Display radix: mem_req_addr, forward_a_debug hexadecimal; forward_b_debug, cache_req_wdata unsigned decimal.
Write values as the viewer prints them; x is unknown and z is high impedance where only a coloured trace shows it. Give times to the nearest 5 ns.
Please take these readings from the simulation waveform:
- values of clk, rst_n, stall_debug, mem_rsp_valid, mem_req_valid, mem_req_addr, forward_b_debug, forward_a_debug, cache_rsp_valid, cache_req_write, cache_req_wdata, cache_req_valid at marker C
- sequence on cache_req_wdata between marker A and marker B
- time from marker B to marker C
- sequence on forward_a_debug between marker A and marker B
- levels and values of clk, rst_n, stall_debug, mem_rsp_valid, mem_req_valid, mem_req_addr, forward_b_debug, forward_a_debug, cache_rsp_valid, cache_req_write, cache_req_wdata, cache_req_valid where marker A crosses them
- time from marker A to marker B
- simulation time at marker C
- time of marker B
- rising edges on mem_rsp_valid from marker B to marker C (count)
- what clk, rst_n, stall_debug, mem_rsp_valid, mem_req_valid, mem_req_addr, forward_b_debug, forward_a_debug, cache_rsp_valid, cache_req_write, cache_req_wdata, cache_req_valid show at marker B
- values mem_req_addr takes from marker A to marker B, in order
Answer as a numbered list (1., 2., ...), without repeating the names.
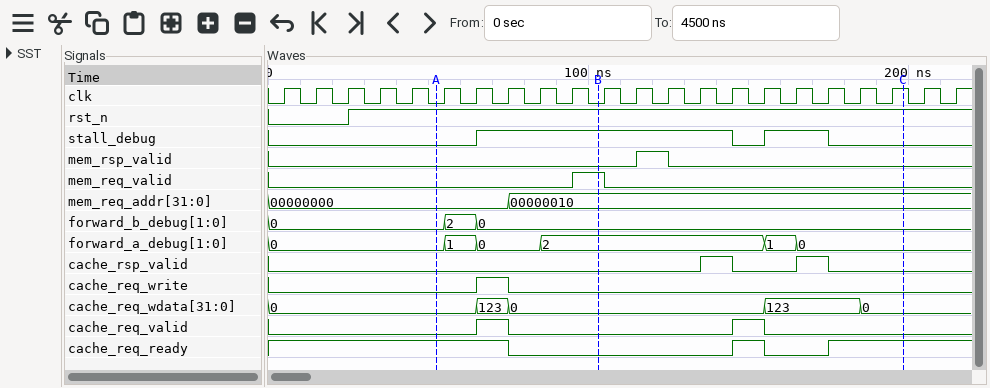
1. clk=1, rst_n=1, stall_debug=0, mem_rsp_valid=0, mem_req_valid=0, mem_req_addr=00000010, forward_b_debug=0, forward_a_debug=0, cache_rsp_valid=0, cache_req_write=0, cache_req_wdata=0, cache_req_valid=0
2. 0, 123, 0
3. 95 ns
4. 0, 1, 0, 2
5. clk=0, rst_n=1, stall_debug=0, mem_rsp_valid=0, mem_req_valid=0, mem_req_addr=00000000, forward_b_debug=0, forward_a_debug=0, cache_rsp_valid=0, cache_req_write=0, cache_req_wdata=0, cache_req_valid=0
6. 50 ns
7. 200 ns
8. 105 ns
9. 1
10. clk=0, rst_n=1, stall_debug=1, mem_rsp_valid=0, mem_req_valid=1, mem_req_addr=00000010, forward_b_debug=0, forward_a_debug=2, cache_rsp_valid=0, cache_req_write=0, cache_req_wdata=0, cache_req_valid=0
11. 00000000, 00000010
